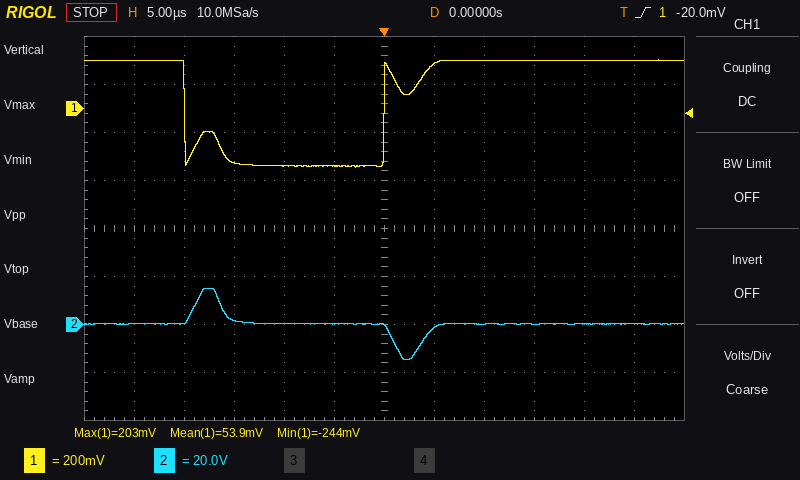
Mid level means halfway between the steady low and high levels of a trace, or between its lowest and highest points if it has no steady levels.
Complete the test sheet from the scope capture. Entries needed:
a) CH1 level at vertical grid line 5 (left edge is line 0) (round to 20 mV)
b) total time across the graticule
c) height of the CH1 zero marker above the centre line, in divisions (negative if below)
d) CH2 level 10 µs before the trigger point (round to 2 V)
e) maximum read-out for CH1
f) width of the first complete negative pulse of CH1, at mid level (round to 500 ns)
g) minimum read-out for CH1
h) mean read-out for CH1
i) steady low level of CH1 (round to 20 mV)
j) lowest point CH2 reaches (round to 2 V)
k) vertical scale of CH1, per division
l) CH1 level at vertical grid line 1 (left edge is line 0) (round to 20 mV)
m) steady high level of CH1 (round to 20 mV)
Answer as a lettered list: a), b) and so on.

a) -240 mV
b) 60 µs
c) +2.5 div
d) 0 V
e) 203 mV
f) 20.0 µs
g) -244 mV
h) 53.9 mV
i) -240 mV
j) -14 V
k) 200 mV
l) 200 mV
m) 200 mV
